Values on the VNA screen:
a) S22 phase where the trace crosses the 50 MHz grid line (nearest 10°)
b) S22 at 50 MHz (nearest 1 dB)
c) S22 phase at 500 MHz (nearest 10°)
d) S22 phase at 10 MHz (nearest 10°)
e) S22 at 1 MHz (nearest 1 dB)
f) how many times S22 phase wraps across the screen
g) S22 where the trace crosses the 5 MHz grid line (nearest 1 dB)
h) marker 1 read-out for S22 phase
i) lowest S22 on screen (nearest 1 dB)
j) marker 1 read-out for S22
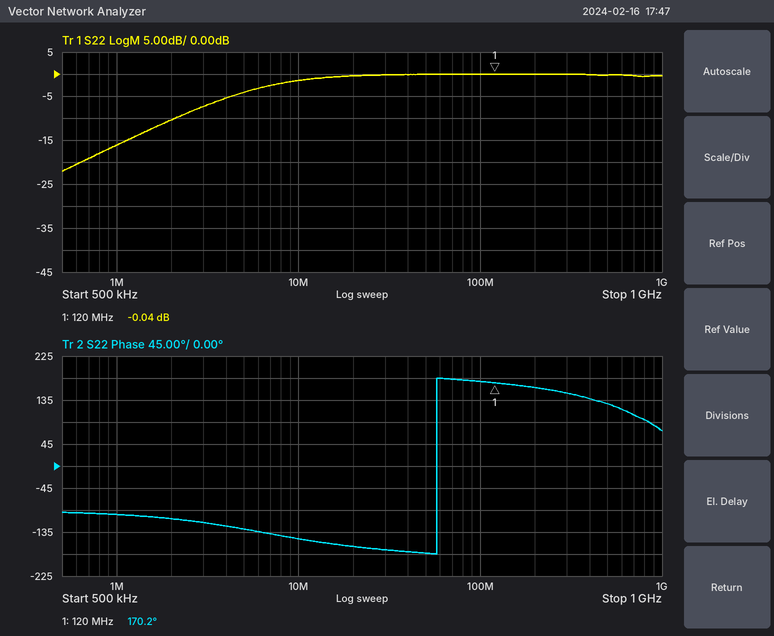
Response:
-180°
0 dB
130°
-150°
-16 dB
1
-4 dB
170.2°
-22 dB
-0.04 dB
